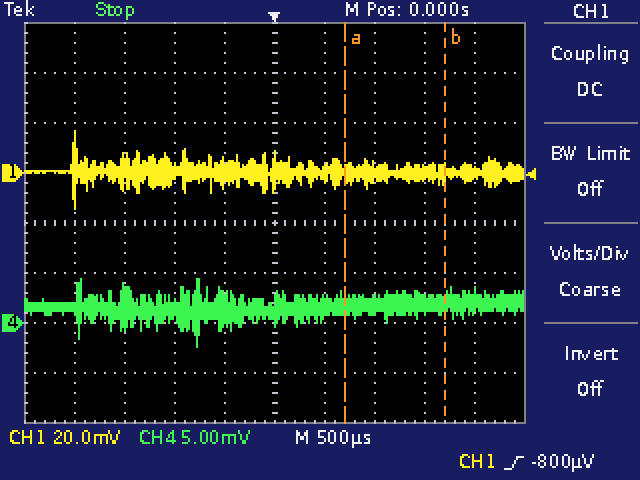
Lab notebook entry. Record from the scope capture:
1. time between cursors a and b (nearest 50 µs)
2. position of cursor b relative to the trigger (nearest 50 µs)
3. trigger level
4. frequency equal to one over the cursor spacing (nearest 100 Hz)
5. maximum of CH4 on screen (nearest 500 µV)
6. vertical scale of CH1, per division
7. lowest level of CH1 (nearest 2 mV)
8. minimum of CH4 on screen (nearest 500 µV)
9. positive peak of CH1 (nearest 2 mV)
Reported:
1.00 ms
+1.70 ms
-800 µV
1.0 kHz
4.5 mV
20 mV
-14 mV
-2.5 mV
16 mV
